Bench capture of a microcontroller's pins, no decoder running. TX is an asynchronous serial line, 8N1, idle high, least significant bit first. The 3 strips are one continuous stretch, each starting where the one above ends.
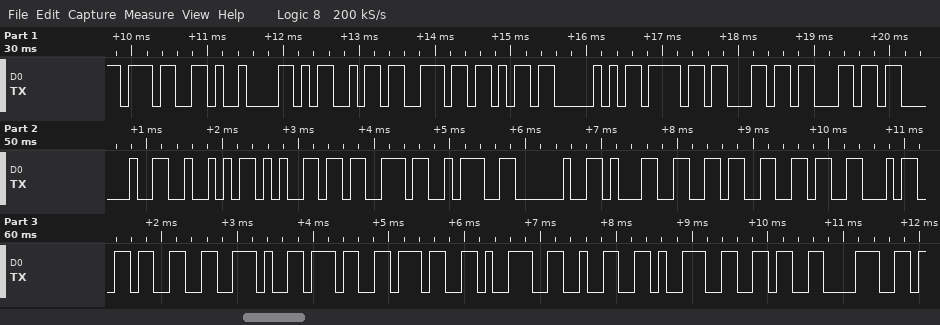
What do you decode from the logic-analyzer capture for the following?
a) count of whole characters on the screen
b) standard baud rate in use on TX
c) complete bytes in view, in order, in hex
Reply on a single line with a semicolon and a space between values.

28; 9600 baud; 0x37 0x09 0x4D 0x73 0x6B 0x50 0x6F 0x6C 0x6C 0x20 0x52 0x65 0x73 0x3A 0x20 0x31 0x36 0x36 0x34 0x33 0x2E 0x37 0x37 0x39 0x32 0x39 0x36 0x38
